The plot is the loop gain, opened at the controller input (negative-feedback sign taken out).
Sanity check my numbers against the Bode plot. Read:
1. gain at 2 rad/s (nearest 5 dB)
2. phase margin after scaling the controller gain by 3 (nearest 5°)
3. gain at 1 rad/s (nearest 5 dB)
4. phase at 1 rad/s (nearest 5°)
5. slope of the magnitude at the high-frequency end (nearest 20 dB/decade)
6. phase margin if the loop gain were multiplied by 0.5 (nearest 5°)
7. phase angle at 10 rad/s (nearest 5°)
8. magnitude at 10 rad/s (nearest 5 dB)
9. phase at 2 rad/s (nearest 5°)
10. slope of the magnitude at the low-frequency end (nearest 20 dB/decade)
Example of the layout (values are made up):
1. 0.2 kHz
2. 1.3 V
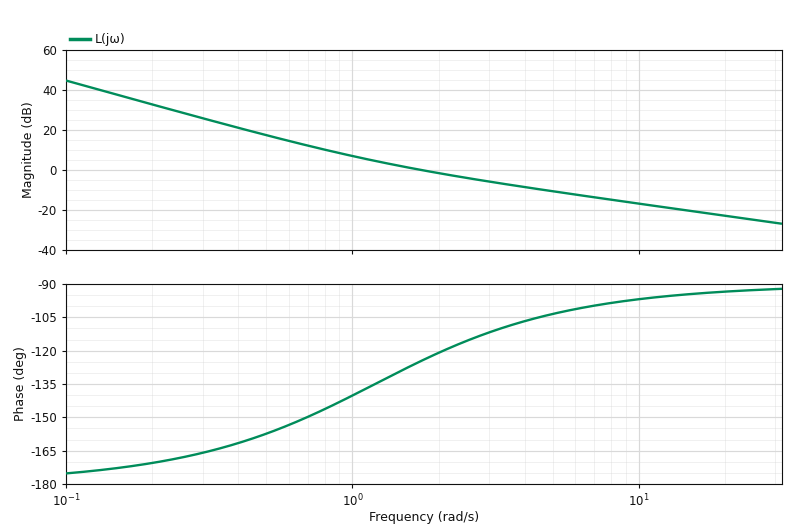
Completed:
1. 0 dB
2. 75°
3. 5 dB
4. -140°
5. -20 dB/decade
6. 40°
7. -95°
8. -15 dB
9. -120°
10. -40 dB/decade
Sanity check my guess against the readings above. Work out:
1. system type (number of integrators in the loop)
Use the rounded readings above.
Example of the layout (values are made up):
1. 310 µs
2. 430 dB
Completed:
1. 2
